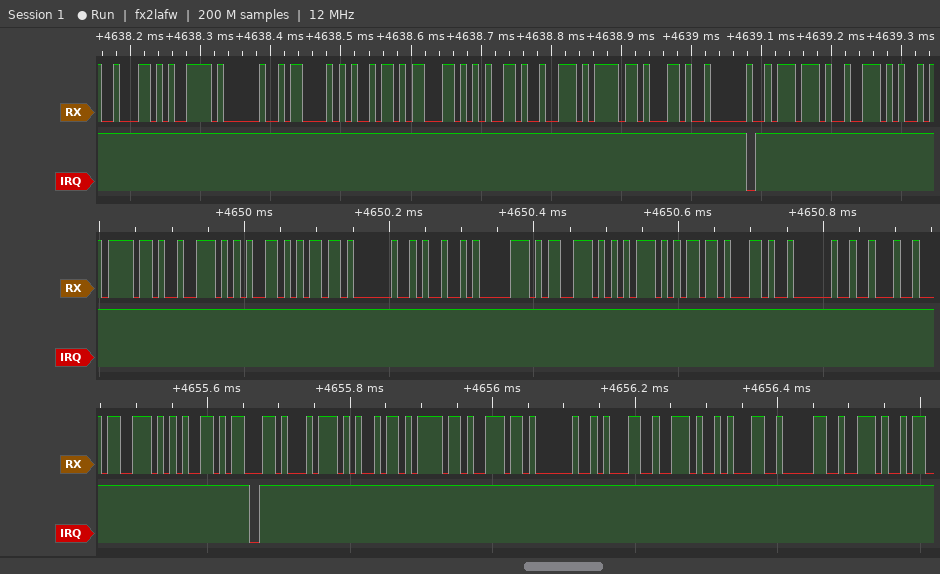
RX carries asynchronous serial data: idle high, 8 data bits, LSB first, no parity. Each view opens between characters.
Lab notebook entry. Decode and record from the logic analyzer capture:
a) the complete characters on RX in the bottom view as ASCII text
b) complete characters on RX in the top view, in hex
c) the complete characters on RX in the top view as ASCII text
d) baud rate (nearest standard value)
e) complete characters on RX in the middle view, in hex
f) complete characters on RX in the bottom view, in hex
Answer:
"section 1.10."
62, 79, 20, 43, 69, 63, 65, 72, 6F, 2C, 20, 77, 72
"by Cicero, wr"
115200 baud
6F, 72, 65, 6D, 20, 49, 70, 73, 75, 6D, 2C, 20, 22
73, 65, 63, 74, 69, 6F, 6E, 20, 31, 2E, 31, 30, 2E
